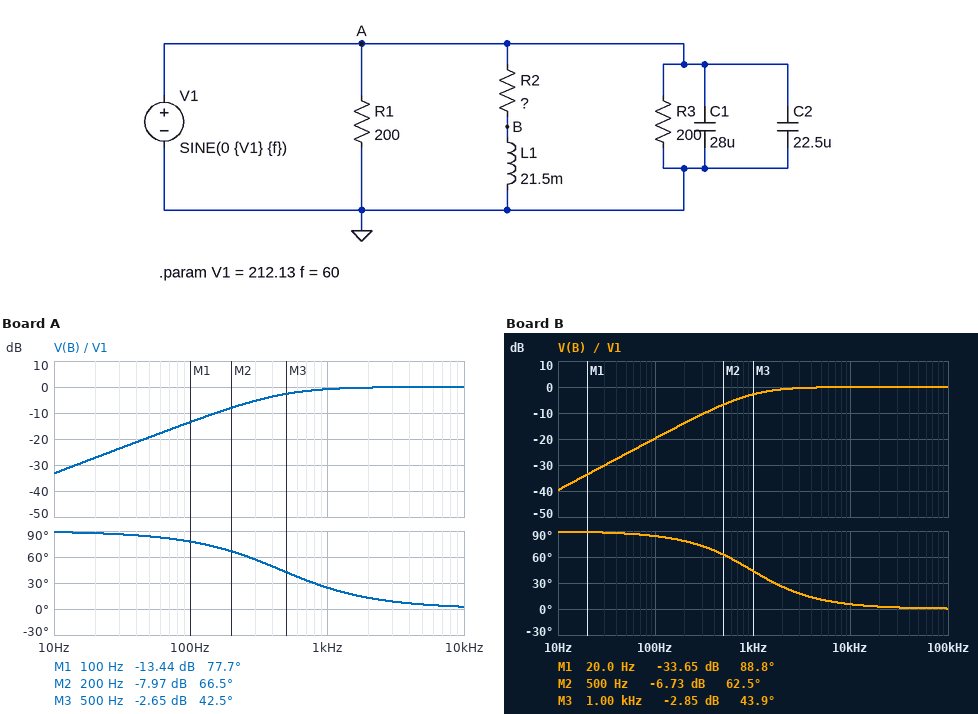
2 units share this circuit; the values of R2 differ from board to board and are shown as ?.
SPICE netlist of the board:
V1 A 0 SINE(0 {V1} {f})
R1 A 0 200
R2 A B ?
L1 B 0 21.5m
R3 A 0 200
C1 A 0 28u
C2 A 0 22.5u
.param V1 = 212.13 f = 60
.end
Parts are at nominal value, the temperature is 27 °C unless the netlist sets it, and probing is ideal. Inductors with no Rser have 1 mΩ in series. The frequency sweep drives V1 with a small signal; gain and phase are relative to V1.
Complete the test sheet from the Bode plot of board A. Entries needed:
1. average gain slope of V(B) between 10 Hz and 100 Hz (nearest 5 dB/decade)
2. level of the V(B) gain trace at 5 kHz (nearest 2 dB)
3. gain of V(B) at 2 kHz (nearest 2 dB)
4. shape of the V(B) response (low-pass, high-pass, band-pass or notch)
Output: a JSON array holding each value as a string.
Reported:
["20 dB/decade", "0 dB", "0 dB", "high-pass"]
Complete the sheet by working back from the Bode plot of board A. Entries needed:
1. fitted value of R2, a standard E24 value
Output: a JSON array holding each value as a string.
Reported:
["62 Ω"]
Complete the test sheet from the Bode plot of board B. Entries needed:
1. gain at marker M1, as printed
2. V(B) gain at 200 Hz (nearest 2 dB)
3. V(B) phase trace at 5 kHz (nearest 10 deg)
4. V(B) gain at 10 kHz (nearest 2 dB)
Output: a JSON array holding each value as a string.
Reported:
["-33.65 dB", "-14 dB", "10 deg", "0 dB"]
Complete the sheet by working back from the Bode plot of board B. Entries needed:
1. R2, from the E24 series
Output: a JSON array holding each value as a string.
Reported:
["130 Ω"]
